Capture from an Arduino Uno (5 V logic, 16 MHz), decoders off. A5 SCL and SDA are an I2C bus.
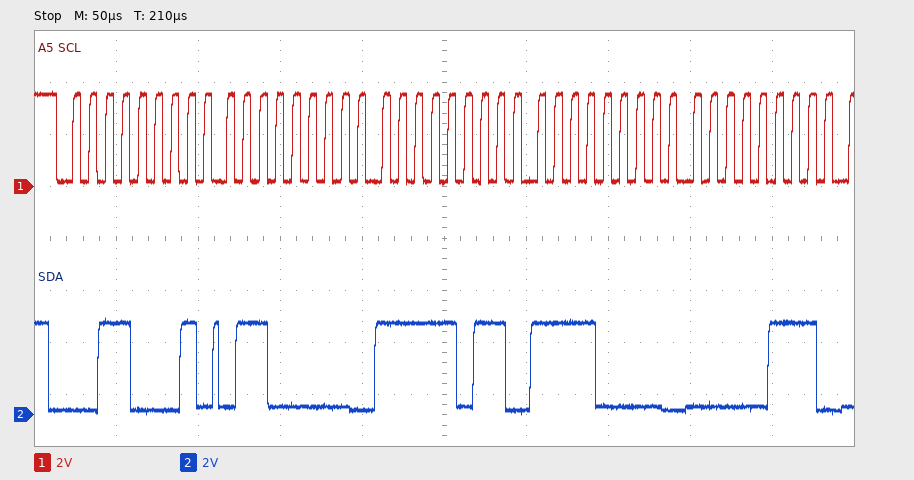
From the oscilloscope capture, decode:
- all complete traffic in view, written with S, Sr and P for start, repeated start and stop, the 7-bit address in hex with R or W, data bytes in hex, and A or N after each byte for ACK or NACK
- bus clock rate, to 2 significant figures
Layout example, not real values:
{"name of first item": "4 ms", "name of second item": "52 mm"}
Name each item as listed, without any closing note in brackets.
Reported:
{"all complete traffic in view, written with S, Sr and P for start, repeated start and stop, the 7-bit address in hex with R or W, data bytes in hex, and A or N after each byte for ACK or NACK": "S 18R A 60 A FB A F0 A 07 A", "bus clock rate, to 2 significant figures": "100 kHz"}
